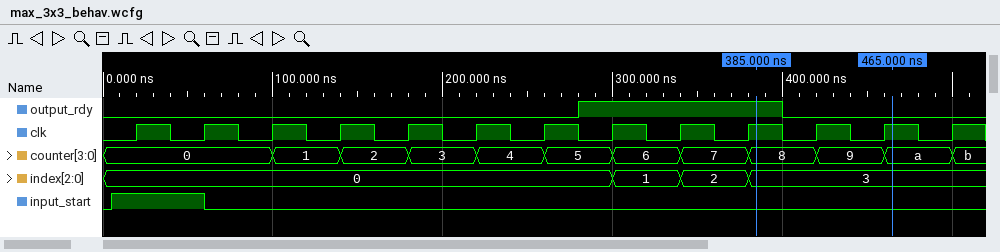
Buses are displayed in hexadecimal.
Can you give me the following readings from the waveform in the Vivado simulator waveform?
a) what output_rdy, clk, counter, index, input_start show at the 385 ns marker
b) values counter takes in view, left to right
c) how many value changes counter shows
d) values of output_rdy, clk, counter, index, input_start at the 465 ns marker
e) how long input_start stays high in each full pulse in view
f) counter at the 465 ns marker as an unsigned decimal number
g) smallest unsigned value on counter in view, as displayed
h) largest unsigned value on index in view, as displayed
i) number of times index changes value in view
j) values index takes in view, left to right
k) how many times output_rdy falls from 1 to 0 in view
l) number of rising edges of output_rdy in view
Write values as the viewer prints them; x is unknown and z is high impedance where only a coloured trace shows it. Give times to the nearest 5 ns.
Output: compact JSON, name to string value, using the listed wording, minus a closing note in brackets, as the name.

{"what output_rdy, clk, counter, index, input_start show at the 385 ns marker": "output_rdy=1, clk=1, counter=8, index=3, input_start=0", "values counter takes in view, left to right": "0, 1, 2, 3, 4, 5, 6, 7, 8, 9, a, b", "how many value changes counter shows": "11", "values of output_rdy, clk, counter, index, input_start at the 465 ns marker": "output_rdy=0, clk=1, counter=a, index=3, input_start=0", "how long input_start stays high in each full pulse in view": "55 ns", "counter at the 465 ns marker as an unsigned decimal number": "10", "smallest unsigned value on counter in view, as displayed": "0", "largest unsigned value on index in view, as displayed": "3", "number of times index changes value in view": "3", "values index takes in view, left to right": "0, 1, 2, 3", "how many times output_rdy falls from 1 to 0 in view": "1", "number of rising edges of output_rdy in view": "1"}
